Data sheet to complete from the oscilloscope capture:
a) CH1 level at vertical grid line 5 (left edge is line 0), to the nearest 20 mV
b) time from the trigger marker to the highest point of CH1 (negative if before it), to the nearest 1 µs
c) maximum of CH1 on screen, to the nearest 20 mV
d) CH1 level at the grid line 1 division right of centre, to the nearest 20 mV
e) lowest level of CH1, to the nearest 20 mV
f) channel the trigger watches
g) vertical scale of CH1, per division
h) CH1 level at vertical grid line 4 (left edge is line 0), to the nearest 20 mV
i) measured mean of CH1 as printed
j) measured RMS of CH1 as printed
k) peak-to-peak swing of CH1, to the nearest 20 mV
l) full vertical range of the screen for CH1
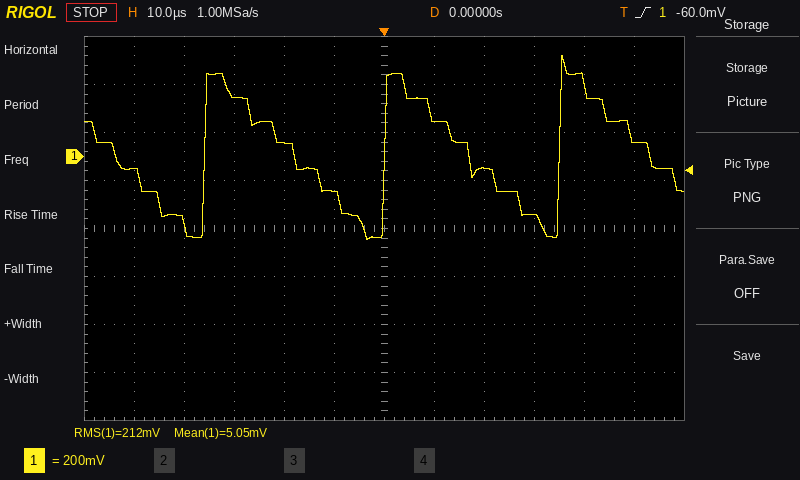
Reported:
-140 mV
+36 µs
420 mV
160 mV
-340 mV
CH1
200 mV
60 mV
5.05 mV
212 mV
760 mV
1.6 V
